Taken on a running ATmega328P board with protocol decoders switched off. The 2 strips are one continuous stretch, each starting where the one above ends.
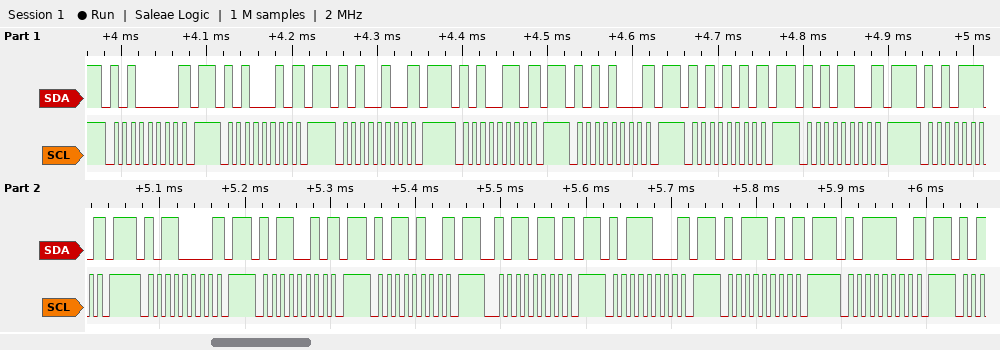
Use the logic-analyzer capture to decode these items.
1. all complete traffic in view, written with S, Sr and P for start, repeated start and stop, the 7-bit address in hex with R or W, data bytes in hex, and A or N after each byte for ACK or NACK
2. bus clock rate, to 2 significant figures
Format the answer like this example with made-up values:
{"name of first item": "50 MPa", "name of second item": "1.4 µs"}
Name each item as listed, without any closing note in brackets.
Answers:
{"all complete traffic in view, written with S, Sr and P for start, repeated start and stop, the 7-bit address in hex with R or W, data bytes in hex, and A or N after each byte for ACK or NACK": "S 50W N P S 51W N P S 52W N P S 53W N P S 54W N P S 55W N P S 56W N P S 57W N P S 58W N P S 59W N P S 5AW N P S 5BW N P S 5CW N P S 5DW N P S 5EW N P", "bus clock rate, to 2 significant figures": "100 kHz"}
